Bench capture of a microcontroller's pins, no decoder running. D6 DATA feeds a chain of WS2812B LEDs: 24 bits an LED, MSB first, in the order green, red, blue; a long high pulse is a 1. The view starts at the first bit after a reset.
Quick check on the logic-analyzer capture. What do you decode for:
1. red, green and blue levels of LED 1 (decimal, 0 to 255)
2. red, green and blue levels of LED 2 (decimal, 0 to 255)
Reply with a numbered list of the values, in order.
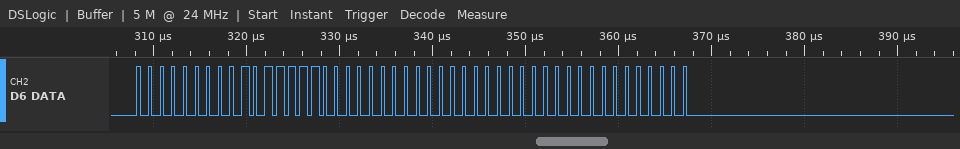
1. 95, 0, 0
2. 0, 0, 0
